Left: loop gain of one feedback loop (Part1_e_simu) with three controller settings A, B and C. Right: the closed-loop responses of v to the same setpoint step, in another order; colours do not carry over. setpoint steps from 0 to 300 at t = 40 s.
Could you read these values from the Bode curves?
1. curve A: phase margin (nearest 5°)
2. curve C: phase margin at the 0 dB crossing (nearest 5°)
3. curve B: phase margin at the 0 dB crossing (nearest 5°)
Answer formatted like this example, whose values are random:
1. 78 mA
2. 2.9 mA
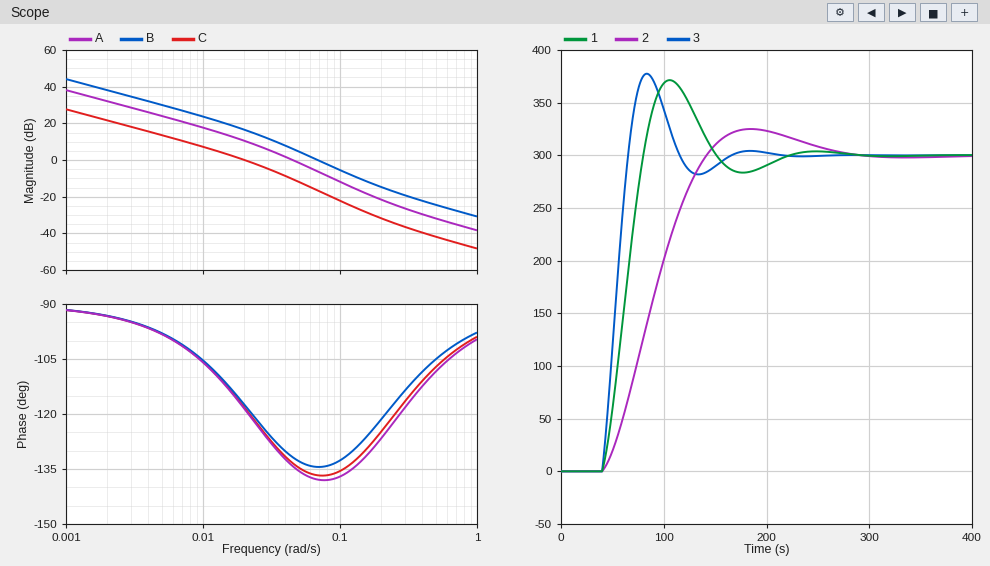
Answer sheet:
1. 45°
2. 60°
3. 45°
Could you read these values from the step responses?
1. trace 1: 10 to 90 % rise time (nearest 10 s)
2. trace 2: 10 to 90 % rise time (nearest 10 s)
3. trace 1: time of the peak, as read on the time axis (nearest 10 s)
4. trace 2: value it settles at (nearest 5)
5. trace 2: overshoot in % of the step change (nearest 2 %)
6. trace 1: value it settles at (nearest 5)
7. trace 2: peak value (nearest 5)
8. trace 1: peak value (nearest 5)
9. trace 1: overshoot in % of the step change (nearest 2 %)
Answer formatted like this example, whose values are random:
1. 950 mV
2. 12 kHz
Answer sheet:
1. 30 s
2. 70 s
3. 110 s
4. 300
5. 8 %
6. 300
7. 325
8. 370
9. 24 %
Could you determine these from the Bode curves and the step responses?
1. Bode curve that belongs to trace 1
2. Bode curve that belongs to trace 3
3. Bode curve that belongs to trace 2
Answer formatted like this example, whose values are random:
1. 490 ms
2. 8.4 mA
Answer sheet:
1. A
2. B
3. C
